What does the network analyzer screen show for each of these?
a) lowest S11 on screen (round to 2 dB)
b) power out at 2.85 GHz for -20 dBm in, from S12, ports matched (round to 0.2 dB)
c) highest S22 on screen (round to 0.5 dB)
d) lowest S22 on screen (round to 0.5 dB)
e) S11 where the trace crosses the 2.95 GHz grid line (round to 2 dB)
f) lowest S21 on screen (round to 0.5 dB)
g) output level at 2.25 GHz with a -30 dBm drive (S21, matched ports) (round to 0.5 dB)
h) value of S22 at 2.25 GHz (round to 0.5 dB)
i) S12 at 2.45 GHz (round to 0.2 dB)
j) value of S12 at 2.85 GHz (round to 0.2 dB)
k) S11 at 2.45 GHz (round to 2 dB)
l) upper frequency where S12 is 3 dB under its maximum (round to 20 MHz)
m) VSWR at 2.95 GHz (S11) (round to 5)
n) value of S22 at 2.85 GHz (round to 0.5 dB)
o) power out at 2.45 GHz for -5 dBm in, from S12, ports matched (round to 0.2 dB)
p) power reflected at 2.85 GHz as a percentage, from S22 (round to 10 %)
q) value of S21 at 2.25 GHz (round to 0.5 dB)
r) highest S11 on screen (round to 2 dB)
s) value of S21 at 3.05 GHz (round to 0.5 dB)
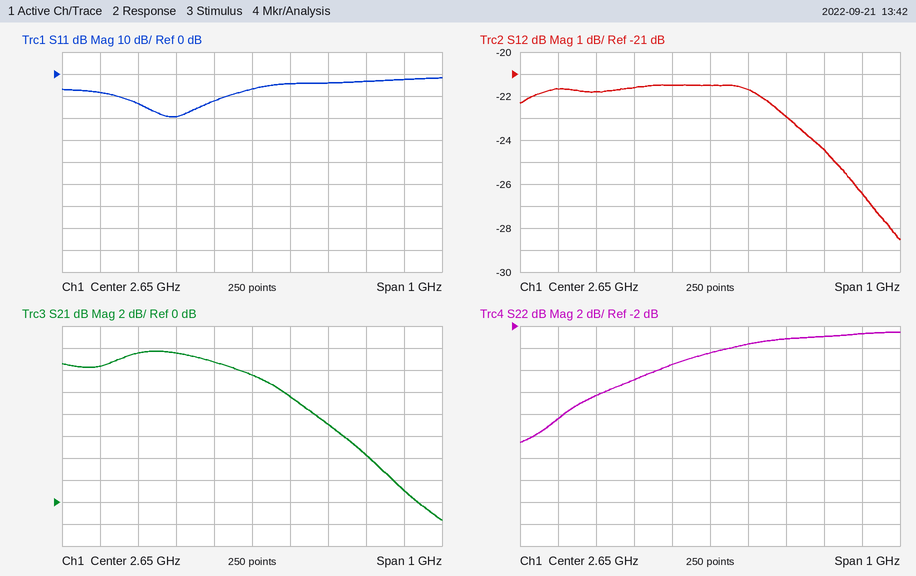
-20 dB
-43.0 dBm
-2.5 dB
-12.5 dB
-4 dB
-1.5 dB
-17.5 dBm
-10.5 dB
-21.6 dB
-23.0 dB
-20 dB
2.96 GHz
5
-3.0 dB
-26.6 dBm
50 %
12.5 dB
-2 dB
1.0 dB
